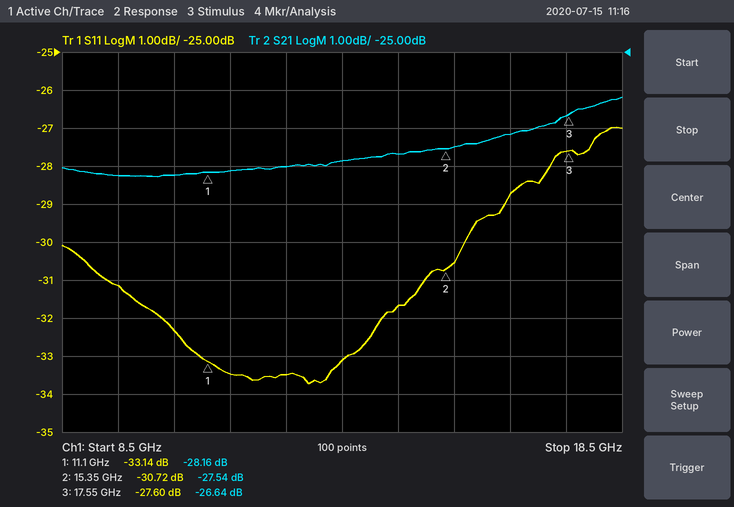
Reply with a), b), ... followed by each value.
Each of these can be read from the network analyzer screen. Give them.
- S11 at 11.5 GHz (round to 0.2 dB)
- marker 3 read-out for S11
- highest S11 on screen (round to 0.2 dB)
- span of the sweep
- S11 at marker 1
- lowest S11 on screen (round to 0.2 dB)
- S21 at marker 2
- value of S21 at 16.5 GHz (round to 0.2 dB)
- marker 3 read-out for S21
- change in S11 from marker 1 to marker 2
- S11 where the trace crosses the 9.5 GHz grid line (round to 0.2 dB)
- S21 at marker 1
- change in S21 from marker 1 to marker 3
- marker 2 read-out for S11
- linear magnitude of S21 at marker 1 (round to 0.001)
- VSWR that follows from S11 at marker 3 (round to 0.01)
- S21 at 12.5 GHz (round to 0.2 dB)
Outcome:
a) -33.4 dB
b) -27.60 dB
c) -27.0 dB
d) 10 GHz
e) -33.14 dB
f) -33.8 dB
g) -27.54 dB
h) -27.2 dB
i) -26.64 dB
j) 2.42 dB
k) -31.2 dB
l) -28.16 dB
m) 1.52 dB
n) -30.72 dB
o) 0.039
p) 1.09
q) -28.0 dB
